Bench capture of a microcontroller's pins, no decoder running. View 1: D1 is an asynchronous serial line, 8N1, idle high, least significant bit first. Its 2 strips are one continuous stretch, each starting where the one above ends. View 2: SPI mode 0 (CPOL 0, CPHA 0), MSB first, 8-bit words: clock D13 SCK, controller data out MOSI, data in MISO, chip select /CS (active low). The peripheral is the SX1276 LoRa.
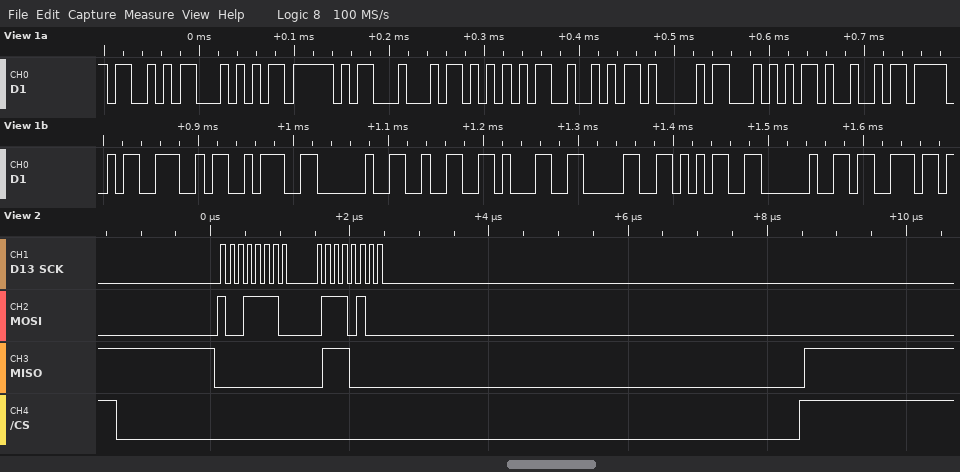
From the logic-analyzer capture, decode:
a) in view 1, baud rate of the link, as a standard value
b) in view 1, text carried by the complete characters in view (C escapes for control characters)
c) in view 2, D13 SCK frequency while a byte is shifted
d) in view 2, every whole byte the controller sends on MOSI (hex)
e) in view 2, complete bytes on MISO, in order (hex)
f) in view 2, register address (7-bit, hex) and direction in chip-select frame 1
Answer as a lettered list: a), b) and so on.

a) 115200 baud
b) "ST_DURATION: 2105 s"
c) 8 MHz
d) 9E 74
e) 00 70
f) 0x1E write
